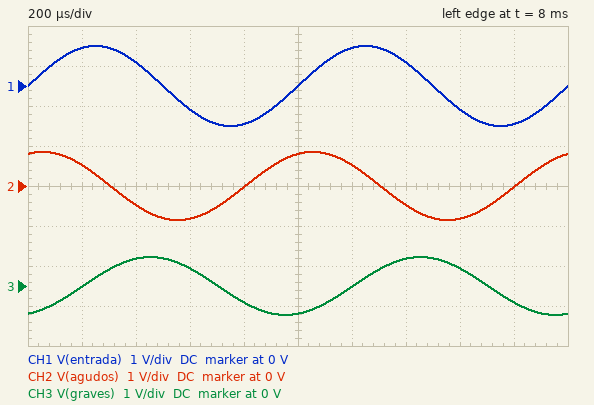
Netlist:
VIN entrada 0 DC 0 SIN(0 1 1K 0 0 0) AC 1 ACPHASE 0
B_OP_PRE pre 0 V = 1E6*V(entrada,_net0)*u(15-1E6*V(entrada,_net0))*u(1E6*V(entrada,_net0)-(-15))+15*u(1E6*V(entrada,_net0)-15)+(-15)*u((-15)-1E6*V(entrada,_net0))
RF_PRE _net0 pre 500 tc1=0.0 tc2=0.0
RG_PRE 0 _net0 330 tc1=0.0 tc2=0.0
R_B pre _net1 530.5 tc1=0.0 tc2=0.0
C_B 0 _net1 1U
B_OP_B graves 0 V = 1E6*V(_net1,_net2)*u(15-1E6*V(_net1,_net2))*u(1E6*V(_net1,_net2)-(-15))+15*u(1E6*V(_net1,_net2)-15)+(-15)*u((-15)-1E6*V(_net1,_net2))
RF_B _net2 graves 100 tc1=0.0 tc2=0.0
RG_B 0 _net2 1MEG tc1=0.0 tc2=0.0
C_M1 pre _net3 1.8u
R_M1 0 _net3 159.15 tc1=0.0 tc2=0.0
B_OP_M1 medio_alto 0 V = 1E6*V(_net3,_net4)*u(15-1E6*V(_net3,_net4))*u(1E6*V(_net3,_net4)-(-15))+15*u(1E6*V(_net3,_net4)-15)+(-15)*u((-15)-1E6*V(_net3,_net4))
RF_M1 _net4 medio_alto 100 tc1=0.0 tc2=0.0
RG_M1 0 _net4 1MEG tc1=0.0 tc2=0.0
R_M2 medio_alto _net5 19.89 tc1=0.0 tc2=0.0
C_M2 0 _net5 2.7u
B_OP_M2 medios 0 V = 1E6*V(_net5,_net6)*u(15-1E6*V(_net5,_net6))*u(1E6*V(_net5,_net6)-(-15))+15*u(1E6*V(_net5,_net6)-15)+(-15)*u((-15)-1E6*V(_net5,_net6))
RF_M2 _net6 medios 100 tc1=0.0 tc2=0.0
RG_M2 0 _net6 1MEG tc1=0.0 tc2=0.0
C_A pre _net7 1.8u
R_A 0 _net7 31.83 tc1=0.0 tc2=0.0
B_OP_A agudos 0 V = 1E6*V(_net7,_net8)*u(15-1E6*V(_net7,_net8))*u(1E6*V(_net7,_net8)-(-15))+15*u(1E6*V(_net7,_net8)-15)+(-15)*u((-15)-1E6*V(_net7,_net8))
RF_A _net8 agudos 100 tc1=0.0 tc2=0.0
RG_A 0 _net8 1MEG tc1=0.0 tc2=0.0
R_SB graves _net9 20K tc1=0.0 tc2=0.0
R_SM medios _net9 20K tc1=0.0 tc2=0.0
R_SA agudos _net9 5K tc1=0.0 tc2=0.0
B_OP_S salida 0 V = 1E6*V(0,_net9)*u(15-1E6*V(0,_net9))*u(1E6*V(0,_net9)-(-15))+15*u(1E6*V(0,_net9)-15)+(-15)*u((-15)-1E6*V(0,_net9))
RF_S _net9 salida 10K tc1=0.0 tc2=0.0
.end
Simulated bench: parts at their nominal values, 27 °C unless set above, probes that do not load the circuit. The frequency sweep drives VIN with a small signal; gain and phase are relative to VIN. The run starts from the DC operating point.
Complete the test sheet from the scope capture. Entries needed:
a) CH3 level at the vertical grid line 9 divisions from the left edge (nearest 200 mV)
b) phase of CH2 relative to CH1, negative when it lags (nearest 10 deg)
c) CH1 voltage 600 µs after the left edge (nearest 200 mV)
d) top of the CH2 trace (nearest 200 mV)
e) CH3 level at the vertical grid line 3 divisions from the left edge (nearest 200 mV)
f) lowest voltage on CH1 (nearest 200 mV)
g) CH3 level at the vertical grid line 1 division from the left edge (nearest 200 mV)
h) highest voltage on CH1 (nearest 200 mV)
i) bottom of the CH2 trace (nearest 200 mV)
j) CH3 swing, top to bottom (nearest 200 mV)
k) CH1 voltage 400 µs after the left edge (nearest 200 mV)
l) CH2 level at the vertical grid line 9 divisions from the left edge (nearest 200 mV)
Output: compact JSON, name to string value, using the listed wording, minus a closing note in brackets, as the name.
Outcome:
{"CH3 level at the vertical grid line 9 divisions from the left edge": "-400 mV", "phase of CH2 relative to CH1, negative when it lags": "70 deg", "CH1 voltage 600 µs after the left edge": "-600 mV", "top of the CH2 trace": "800 mV", "CH3 level at the vertical grid line 3 divisions from the left edge": "400 mV", "lowest voltage on CH1": "-1.0 V", "CH3 level at the vertical grid line 1 division from the left edge": "0 V", "highest voltage on CH1": "1.0 V", "bottom of the CH2 trace": "-800 mV", "CH3 swing, top to bottom": "1.4 V", "CH1 voltage 400 µs after the left edge": "600 mV", "CH2 level at the vertical grid line 9 divisions from the left edge": "0 V"}
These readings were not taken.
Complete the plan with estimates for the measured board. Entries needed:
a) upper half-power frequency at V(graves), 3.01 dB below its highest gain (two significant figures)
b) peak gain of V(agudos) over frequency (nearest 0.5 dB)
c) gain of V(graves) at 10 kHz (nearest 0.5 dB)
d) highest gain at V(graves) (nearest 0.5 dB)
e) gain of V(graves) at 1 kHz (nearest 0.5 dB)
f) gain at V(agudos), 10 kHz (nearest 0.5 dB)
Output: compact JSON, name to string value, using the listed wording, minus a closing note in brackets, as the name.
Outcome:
{"upper half-power frequency at V(graves), 3.01 dB below its highest gain": "300 Hz", "peak gain of V(agudos) over frequency": "8.0 dB", "gain of V(graves) at 10 kHz": "-22.5 dB", "highest gain at V(graves)": "8.0 dB", "gain of V(graves) at 1 kHz": "-3.0 dB", "gain at V(agudos), 10 kHz": "7.5 dB"}
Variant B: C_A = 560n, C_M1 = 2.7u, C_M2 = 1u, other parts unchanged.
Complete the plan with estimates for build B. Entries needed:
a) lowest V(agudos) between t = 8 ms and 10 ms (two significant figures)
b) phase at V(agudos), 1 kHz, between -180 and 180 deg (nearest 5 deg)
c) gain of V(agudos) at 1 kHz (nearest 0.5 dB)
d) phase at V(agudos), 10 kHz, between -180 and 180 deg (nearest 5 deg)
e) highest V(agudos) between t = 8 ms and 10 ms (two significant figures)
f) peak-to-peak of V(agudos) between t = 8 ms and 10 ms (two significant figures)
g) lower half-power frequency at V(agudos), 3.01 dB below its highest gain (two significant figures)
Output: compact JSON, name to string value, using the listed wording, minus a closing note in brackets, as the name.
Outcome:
{"lowest V(agudos) between t = 8 ms and 10 ms": "-280 mV", "phase at V(agudos), 1 kHz, between -180 and 180 deg": "85 deg", "gain of V(agudos) at 1 kHz": "-11.0 dB", "phase at V(agudos), 10 kHz, between -180 and 180 deg": "40 deg", "highest V(agudos) between t = 8 ms and 10 ms": "280 mV", "peak-to-peak of V(agudos) between t = 8 ms and 10 ms": "560 mV", "lower half-power frequency at V(agudos), 3.01 dB below its highest gain": "8.9 kHz"}
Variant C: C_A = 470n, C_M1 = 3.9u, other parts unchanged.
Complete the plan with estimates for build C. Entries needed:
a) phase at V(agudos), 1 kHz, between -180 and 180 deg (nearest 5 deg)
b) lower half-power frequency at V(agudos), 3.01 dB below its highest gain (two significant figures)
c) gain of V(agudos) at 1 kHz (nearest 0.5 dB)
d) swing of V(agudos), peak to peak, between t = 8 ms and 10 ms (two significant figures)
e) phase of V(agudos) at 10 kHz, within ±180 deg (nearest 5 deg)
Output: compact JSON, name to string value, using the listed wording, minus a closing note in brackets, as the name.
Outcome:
{"phase at V(agudos), 1 kHz, between -180 and 180 deg": "85 deg", "lower half-power frequency at V(agudos), 3.01 dB below its highest gain": "11 kHz", "gain of V(agudos) at 1 kHz": "-12.5 dB", "swing of V(agudos), peak to peak, between t = 8 ms and 10 ms": "470 mV", "phase of V(agudos) at 10 kHz, within ±180 deg": "45 deg"}
